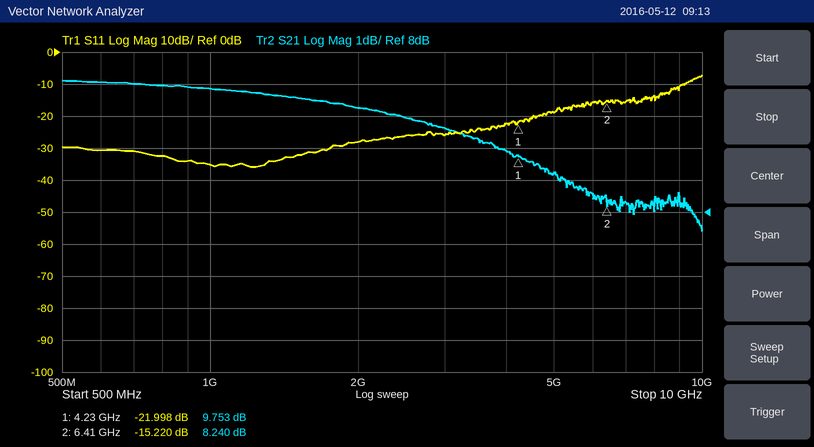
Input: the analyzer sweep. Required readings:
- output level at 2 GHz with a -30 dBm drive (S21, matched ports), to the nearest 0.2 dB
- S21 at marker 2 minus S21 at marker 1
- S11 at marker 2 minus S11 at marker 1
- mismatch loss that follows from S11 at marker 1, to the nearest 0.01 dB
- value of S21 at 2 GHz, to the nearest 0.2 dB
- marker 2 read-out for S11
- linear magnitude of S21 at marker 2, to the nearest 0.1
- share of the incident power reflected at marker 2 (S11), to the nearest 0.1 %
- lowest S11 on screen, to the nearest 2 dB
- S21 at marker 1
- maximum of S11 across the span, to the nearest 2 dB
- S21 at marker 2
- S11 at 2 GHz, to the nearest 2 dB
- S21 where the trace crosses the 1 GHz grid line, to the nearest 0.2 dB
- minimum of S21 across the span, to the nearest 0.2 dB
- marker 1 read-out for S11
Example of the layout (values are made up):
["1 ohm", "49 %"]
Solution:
["-18.8 dBm", "-1.513 dB", "6.778 dB", "0.03 dB", "11.2 dB", "-15.220 dB", "2.6", "3.0 %", "-36 dB", "9.753 dB", "-8 dB", "8.240 dB", "-28 dB", "11.8 dB", "7.4 dB", "-21.998 dB"]
